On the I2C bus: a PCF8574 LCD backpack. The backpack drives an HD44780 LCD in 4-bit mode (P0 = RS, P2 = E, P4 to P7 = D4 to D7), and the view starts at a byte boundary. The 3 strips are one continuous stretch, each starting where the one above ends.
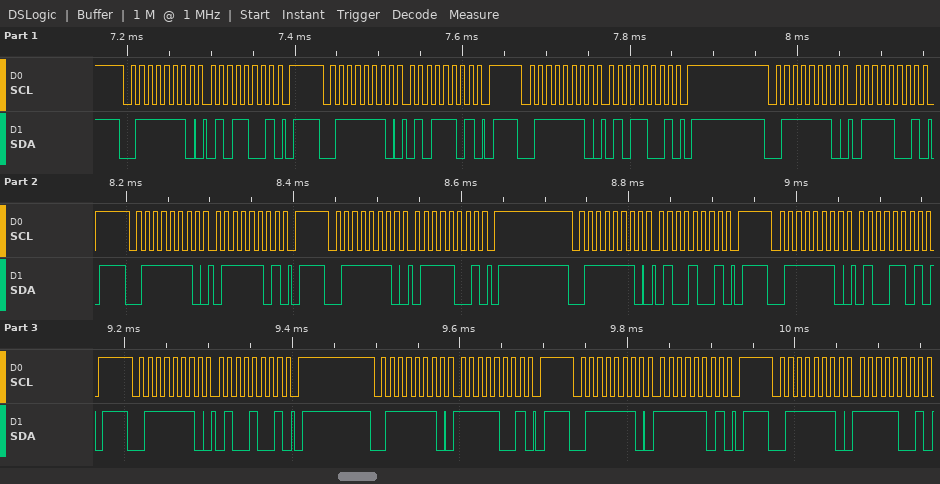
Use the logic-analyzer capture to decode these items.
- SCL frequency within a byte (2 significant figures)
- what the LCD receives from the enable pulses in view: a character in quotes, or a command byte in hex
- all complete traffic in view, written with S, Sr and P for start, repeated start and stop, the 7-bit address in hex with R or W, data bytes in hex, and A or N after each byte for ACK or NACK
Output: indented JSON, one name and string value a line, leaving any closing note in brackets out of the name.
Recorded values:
{
  "SCL frequency within a byte": "100 kHz",
  "what the LCD receives from the enable pulses in view: a character in quotes, or a command byte in hex": "'W' 'O'",
  "all complete traffic in view, written with S, Sr and P for start, repeated start and stop, the 7-bit address in hex with R or W, data bytes in hex, and A or N after each byte for ACK or NACK": "S 3FW A 59 A P S 3FW A 5D A P S 3FW A 59 A P S 3FW A 79 A P S 3FW A 7D A P S 3FW A 79 A P S 3FW A 49 A P S 3FW A 4D A P S 3FW A 49 A P S 3FW A F9 A P S 3FW A FD A P S 3FW A F9 A"
}
